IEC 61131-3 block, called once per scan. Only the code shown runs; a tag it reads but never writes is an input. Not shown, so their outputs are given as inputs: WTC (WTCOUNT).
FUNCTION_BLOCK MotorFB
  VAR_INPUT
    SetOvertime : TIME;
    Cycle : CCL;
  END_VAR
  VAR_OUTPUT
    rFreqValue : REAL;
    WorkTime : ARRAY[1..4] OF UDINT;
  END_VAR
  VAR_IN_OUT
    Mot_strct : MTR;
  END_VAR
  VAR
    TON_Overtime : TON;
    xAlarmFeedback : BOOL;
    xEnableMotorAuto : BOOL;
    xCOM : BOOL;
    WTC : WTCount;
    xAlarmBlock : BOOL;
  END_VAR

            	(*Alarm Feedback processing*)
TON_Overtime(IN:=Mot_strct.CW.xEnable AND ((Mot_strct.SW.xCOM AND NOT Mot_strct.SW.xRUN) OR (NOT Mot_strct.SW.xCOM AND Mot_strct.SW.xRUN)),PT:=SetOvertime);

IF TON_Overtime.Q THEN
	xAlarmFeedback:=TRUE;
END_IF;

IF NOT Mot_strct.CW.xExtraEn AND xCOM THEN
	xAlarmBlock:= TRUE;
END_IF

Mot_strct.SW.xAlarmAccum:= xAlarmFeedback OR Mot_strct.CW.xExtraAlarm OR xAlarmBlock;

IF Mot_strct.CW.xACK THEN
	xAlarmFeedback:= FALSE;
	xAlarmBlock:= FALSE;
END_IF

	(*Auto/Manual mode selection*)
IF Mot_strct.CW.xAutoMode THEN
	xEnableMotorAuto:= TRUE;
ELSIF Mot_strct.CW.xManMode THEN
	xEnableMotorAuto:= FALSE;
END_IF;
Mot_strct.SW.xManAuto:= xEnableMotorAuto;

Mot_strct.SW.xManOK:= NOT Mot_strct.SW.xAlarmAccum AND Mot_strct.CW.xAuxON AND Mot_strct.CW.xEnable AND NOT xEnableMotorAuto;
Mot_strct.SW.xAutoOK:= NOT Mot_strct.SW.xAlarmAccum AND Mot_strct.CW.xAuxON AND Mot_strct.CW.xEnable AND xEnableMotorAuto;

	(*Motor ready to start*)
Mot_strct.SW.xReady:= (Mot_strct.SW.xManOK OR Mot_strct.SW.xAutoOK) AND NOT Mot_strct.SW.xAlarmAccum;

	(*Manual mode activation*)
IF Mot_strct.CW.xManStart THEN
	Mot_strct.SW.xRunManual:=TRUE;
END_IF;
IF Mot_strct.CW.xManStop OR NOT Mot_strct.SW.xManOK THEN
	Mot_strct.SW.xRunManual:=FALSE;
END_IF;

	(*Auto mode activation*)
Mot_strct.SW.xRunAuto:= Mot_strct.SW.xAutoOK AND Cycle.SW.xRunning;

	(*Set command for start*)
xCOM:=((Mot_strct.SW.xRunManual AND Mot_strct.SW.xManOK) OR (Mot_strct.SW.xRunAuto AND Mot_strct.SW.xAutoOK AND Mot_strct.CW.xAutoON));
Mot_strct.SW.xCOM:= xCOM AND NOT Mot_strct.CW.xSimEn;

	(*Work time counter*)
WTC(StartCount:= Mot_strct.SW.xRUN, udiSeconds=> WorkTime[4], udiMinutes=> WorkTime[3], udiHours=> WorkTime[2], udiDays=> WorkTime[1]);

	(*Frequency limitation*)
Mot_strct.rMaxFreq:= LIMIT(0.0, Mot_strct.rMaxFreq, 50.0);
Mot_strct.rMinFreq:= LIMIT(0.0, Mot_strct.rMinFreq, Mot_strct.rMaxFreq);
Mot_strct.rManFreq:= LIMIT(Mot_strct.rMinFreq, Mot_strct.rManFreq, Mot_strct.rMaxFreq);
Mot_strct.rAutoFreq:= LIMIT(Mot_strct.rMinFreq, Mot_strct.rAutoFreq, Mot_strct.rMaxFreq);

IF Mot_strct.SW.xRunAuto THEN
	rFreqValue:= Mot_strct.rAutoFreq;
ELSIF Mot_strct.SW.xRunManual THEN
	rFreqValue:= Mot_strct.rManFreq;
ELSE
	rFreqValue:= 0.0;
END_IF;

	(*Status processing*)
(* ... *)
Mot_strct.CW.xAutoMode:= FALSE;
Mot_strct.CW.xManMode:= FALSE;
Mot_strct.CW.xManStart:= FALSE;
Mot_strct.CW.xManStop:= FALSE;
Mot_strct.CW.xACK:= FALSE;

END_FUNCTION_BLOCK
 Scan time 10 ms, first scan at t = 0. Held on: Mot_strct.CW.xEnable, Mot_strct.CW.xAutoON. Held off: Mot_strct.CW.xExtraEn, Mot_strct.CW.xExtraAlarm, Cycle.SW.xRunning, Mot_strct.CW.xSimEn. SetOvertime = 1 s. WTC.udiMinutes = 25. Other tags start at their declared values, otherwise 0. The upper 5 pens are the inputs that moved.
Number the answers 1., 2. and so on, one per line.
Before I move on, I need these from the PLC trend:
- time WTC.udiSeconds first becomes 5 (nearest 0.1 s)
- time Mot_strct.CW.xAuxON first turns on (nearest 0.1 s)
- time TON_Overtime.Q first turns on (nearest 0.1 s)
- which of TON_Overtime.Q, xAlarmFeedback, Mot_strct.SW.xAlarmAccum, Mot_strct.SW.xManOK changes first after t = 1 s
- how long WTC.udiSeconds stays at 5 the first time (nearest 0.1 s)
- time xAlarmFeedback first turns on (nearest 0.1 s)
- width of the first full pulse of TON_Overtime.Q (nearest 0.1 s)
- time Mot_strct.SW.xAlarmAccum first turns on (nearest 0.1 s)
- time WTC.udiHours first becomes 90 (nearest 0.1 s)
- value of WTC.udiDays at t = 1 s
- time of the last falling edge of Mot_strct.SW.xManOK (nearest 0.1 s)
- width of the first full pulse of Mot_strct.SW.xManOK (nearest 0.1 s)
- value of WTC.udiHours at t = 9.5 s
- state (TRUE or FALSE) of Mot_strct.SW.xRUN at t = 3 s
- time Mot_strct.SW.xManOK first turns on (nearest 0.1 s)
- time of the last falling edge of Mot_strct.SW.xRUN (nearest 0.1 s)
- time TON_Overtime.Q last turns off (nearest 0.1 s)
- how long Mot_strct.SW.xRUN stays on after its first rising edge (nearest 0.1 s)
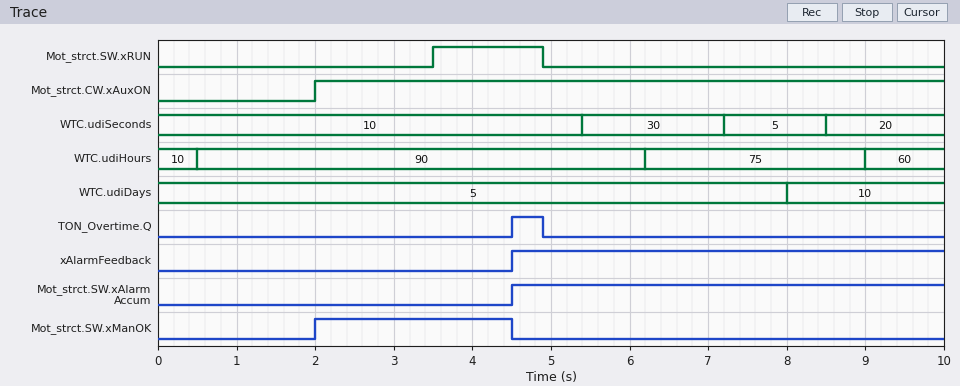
1. 7.2 s
2. 2.0 s
3. 4.5 s
4. Mot_strct.SW.xManOK
5. 1.3 s
6. 4.5 s
7. 0.4 s
8. 4.5 s
9. 0.5 s
10. 5
11. 4.5 s
12. 2.5 s
13. 60
14. FALSE
15. 2.0 s
16. 4.9 s
17. 4.9 s
18. 1.4 s
